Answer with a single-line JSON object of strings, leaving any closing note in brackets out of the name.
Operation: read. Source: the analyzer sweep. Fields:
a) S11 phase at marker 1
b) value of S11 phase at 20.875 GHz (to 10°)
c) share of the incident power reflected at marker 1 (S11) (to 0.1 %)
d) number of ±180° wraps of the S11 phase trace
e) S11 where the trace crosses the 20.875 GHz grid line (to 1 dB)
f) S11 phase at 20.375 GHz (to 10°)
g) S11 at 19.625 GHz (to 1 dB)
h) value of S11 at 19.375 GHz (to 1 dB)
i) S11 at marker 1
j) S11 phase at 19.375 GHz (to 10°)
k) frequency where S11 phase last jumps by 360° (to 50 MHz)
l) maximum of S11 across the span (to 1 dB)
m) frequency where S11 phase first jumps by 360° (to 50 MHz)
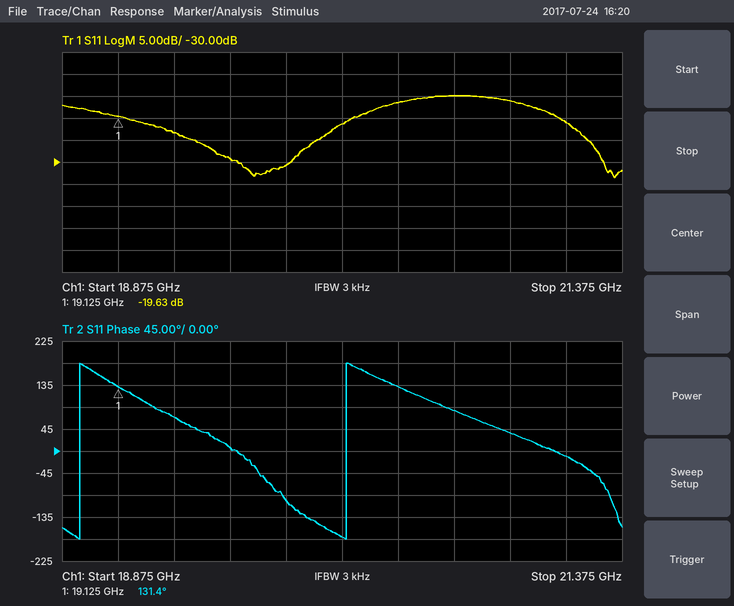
{"S11 phase at marker 1": "131.4°", "value of S11 phase at 20.875 GHz": "40°", "share of the incident power reflected at marker 1 (S11)": "1.1 %", "number of ±180° wraps of the S11 phase trace": "2", "S11 where the trace crosses the 20.875 GHz grid line": "-16 dB", "S11 phase at 20.375 GHz": "130°", "S11 at 19.625 GHz": "-29 dB", "value of S11 at 19.375 GHz": "-23 dB", "S11 at marker 1": "-19.63 dB", "S11 phase at 19.375 GHz": "70°", "frequency where S11 phase last jumps by 360°": "20.15 GHz", "maximum of S11 across the span": "-15 dB", "frequency where S11 phase first jumps by 360°": "18.95 GHz"}
